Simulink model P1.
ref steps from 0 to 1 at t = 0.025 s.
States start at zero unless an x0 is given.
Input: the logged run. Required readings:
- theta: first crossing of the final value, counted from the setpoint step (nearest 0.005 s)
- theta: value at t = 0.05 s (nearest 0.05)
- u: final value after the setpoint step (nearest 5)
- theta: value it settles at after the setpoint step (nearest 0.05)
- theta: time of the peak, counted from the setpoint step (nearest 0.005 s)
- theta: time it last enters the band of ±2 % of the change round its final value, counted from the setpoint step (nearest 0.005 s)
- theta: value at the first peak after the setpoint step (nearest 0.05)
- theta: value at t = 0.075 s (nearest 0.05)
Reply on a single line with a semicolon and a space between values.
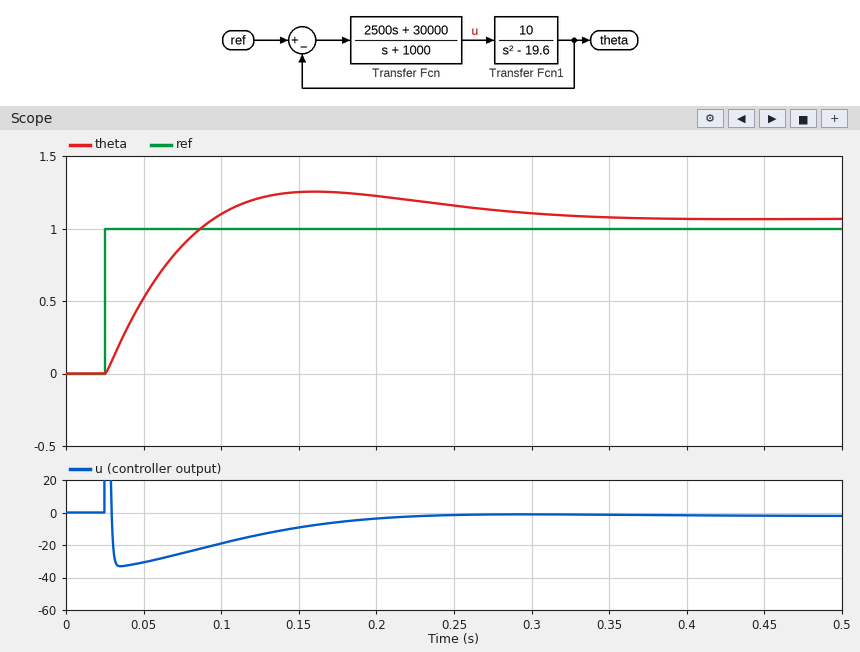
0.070 s; 0.50; 0; 1.05; 0.135 s; 0.295 s; 1.25; 0.90
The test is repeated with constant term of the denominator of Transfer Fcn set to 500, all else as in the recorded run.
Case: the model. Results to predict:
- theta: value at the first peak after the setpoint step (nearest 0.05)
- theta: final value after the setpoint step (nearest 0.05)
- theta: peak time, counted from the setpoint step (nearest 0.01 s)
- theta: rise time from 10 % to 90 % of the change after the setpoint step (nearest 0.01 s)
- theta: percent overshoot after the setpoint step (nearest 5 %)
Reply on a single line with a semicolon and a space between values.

1.15; 1.05; 0.08 s; 0.03 s; 10 %
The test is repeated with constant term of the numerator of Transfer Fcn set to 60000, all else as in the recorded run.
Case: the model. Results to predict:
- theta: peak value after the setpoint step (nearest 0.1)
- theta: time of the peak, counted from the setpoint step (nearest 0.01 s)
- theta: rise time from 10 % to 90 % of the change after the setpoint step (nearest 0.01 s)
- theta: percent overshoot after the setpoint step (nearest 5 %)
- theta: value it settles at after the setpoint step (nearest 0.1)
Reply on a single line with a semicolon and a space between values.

1.3; 0.10 s; 0.04 s; 30 %; 1.0
